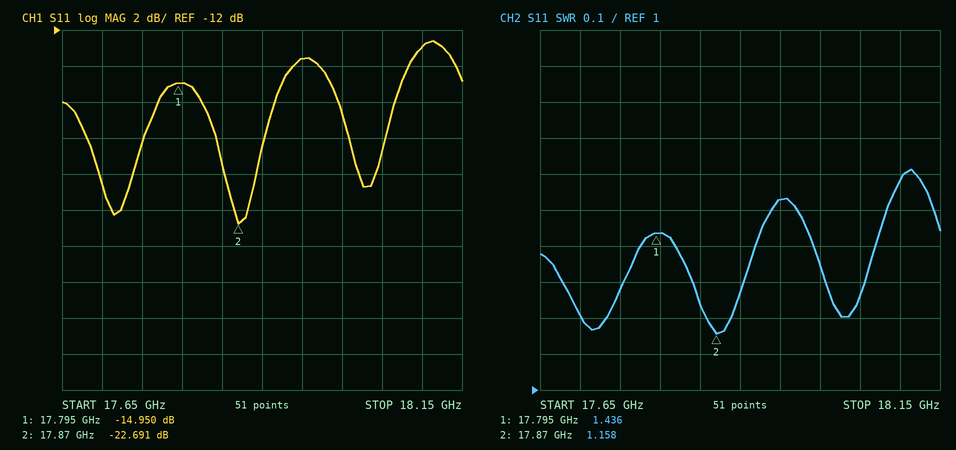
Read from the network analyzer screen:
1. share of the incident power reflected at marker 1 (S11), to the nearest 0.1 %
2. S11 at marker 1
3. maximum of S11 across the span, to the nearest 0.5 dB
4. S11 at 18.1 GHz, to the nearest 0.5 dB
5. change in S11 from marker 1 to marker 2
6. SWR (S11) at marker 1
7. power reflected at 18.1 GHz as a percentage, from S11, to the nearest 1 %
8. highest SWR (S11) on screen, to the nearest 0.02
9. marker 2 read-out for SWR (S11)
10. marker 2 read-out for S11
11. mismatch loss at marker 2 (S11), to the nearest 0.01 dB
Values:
3.2 %
-14.950 dB
-12.5 dB
-13.0 dB
-7.741 dB
1.436
5 %
1.62
1.158
-22.691 dB
0.02 dB
